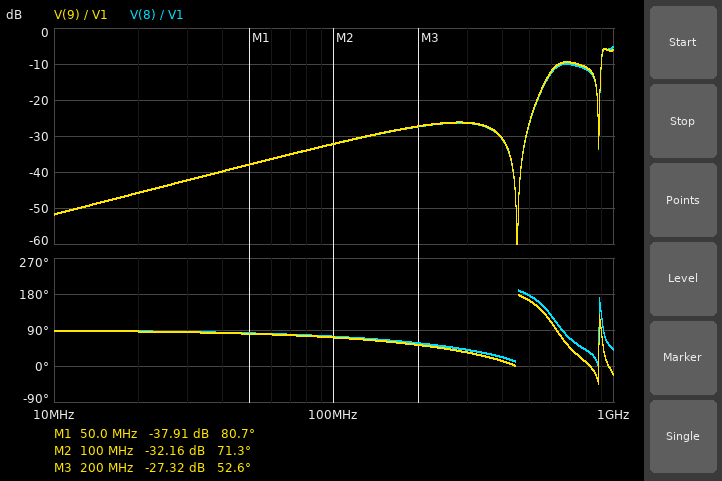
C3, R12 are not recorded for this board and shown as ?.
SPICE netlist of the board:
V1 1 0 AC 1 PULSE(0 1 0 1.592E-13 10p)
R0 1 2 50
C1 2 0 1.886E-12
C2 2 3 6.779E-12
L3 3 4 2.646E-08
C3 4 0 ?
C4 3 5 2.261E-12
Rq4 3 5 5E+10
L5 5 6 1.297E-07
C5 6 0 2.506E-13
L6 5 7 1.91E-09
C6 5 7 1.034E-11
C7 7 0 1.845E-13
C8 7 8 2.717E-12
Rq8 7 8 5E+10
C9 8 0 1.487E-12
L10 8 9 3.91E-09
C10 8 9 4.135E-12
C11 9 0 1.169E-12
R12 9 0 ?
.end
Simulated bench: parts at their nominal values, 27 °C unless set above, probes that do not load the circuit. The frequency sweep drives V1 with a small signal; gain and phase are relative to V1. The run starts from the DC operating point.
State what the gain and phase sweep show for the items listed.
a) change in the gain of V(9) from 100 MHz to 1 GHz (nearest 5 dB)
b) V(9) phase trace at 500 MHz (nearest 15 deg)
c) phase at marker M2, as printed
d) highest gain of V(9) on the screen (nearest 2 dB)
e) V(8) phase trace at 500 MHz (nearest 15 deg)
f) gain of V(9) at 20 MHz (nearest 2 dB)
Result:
25 dB
165 deg
71.3 deg
-6 dB
180 deg
-46 dB
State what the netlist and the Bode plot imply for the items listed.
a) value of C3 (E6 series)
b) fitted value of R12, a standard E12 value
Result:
4.7 pF
68 Ω
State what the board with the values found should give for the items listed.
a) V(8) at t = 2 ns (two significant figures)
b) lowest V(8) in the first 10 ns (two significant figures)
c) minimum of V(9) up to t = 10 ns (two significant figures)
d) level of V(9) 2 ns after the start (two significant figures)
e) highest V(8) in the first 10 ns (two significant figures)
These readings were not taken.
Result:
9.5 mV
-66 mV
-44 mV
-25 mV
130 mV
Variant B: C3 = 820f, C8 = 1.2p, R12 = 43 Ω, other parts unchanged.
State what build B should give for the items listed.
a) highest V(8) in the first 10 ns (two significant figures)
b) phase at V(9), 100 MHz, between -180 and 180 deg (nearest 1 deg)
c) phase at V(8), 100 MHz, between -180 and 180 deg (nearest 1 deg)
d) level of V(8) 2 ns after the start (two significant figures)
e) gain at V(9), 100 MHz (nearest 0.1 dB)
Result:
89 mV
79 deg
82 deg
-5.4 mV
-36.6 dB
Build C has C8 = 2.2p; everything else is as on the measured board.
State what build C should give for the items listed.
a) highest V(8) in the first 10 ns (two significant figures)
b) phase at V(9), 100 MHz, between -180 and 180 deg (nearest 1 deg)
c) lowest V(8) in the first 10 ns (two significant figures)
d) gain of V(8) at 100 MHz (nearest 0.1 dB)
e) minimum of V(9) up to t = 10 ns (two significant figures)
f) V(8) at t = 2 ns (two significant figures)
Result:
120 mV
72 deg
-65 mV
-33.1 dB
-42 mV
11 mV
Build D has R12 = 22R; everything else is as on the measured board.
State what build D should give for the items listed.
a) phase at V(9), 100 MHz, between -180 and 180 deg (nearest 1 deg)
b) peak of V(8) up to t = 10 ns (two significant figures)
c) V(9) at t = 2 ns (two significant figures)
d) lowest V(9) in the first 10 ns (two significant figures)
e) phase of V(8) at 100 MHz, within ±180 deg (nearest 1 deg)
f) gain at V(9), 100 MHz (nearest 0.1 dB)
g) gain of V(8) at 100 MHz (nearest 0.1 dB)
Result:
78 deg
100 mV
-24 mV
-30 mV
84 deg
-41.9 dB
-41.8 dB
